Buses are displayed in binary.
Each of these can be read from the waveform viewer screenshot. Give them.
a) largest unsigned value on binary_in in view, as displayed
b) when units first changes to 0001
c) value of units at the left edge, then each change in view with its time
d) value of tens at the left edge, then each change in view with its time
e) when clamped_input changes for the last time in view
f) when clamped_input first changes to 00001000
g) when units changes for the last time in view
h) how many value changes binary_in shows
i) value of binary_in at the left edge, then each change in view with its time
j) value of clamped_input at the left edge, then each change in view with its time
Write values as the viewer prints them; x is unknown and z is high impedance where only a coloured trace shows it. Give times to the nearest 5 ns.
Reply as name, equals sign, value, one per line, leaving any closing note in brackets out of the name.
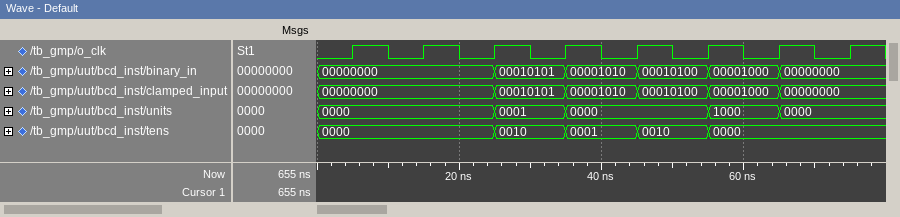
largest unsigned value on binary_in in view, as displayed = 00010101
when units first changes to 0001 = 25 ns
value of units at the left edge, then each change in view with its time = 0000, 0001 at 25 ns, 0000 at 35 ns, 1000 at 55 ns, 0000 at 65 ns
value of tens at the left edge, then each change in view with its time = 0000, 0010 at 25 ns, 0001 at 35 ns, 0010 at 45 ns, 0000 at 55 ns
when clamped_input changes for the last time in view = 65 ns
when clamped_input first changes to 00001000 = 55 ns
when units changes for the last time in view = 65 ns
how many value changes binary_in shows = 5
value of binary_in at the left edge, then each change in view with its time = 00000000, 00010101 at 25 ns, 00001010 at 35 ns, 00010100 at 45 ns, 00001000 at 55 ns, 00000000 at 65 ns
value of clamped_input at the left edge, then each change in view with its time = 00000000, 00010101 at 25 ns, 00001010 at 35 ns, 00010100 at 45 ns, 00001000 at 55 ns, 00000000 at 65 ns
